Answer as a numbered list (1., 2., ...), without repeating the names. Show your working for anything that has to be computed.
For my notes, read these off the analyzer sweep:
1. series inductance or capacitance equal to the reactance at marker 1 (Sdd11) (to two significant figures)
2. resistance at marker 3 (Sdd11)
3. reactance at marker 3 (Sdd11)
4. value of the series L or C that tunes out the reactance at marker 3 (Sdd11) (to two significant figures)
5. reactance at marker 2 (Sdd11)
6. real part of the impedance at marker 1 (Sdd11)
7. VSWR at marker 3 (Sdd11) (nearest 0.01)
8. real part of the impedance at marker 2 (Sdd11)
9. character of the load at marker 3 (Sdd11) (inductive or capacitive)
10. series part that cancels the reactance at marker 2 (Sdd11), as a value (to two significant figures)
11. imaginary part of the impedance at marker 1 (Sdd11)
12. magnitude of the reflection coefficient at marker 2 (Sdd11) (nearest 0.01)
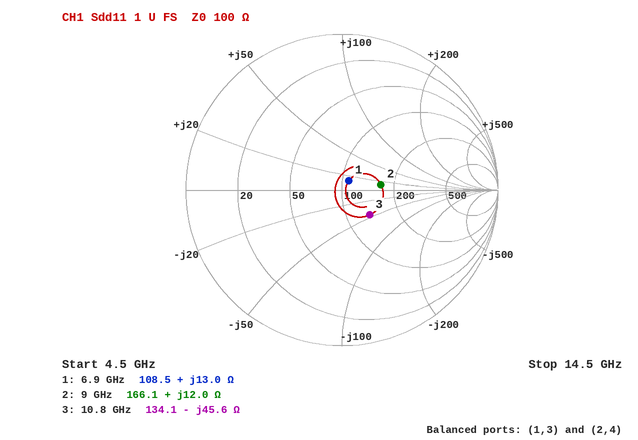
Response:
1. L = 13 Ω/(2π × 6.9 GHz) ≈ 300 pH
2. 134.1 Ω
3. -45.6 Ω
4. L = 45.6 Ω/(2π × 10.8 GHz) ≈ 672 pH, so 670 pH to two significant figures
5. +12.0 Ω
6. 108.5 Ω
7. 1.63
8. 166.1 Ω
9. capacitive
10. C = 1/(2π × 9 GHz × 12 Ω) ≈ 1.5 pF
11. +13.0 Ω
12. 0.25
